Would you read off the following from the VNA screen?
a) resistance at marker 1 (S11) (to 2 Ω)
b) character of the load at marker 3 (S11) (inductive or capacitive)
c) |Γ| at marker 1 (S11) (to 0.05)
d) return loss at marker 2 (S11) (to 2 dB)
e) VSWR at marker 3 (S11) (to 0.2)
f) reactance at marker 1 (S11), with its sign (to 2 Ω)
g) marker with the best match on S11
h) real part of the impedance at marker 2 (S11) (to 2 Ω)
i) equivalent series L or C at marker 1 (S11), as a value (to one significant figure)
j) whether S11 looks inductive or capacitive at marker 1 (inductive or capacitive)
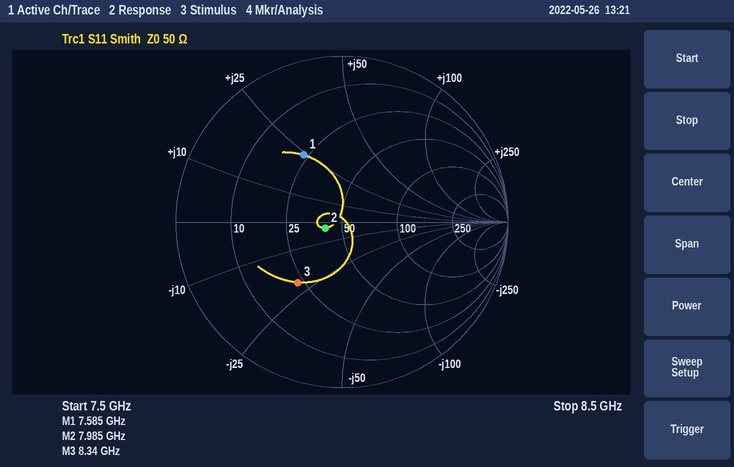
24 Ω
capacitive
0.45
20 dB
2.6
+24 Ω
marker 2
40 Ω
500 pH
inductive
